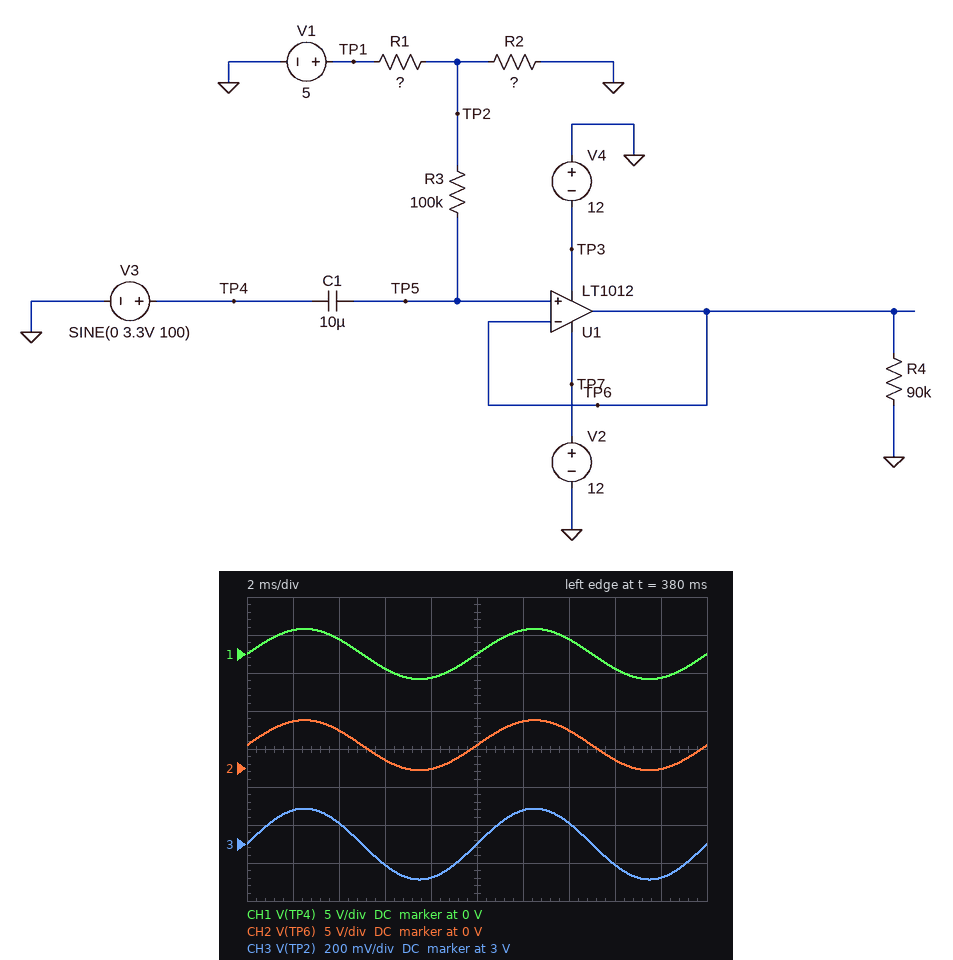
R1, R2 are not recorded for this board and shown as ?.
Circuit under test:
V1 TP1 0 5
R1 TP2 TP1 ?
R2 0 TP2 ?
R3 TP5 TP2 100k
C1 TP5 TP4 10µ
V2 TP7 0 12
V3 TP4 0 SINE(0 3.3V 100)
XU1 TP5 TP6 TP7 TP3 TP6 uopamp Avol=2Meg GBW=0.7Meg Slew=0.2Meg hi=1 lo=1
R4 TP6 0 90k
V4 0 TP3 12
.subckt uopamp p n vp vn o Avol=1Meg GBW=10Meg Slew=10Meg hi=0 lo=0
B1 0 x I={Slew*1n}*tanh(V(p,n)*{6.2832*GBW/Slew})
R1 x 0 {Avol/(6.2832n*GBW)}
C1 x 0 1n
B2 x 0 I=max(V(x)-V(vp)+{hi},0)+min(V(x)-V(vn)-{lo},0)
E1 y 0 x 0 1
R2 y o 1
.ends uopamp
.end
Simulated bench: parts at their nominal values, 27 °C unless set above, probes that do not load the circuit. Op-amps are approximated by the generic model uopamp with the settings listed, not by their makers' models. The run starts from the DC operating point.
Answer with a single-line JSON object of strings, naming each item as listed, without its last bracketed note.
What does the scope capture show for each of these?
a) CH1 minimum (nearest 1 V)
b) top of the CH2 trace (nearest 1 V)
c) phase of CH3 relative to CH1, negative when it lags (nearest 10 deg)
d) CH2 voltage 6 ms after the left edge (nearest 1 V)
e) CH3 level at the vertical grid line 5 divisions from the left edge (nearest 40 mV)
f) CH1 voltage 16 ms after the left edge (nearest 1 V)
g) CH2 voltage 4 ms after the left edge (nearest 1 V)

{"CH1 minimum": "-3 V", "top of the CH2 trace": "6 V", "phase of CH3 relative to CH1, negative when it lags": "0 deg", "CH2 voltage 6 ms after the left edge": "1 V", "CH3 level at the vertical grid line 5 divisions from the left edge": "3.00 V", "CH1 voltage 16 ms after the left edge": "-2 V", "CH2 voltage 4 ms after the left edge": "5 V"}
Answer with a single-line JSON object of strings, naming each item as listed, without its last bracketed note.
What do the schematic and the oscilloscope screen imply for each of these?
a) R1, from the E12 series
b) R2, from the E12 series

{"R1, from the E12 series": "10 kΩ", "R2, from the E12 series": "15 kΩ"}
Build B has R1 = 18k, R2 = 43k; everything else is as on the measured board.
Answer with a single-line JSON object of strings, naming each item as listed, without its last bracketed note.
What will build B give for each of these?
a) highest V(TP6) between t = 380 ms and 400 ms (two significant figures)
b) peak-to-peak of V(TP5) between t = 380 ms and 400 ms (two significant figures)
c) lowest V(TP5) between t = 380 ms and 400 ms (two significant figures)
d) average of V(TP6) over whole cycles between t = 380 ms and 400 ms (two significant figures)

{"highest V(TP6) between t = 380 ms and 400 ms": "6.8 V", "peak-to-peak of V(TP5) between t = 380 ms and 400 ms": "6.6 V", "lowest V(TP5) between t = 380 ms and 400 ms": "220 mV", "average of V(TP6) over whole cycles between t = 380 ms and 400 ms": "3.5 V"}
